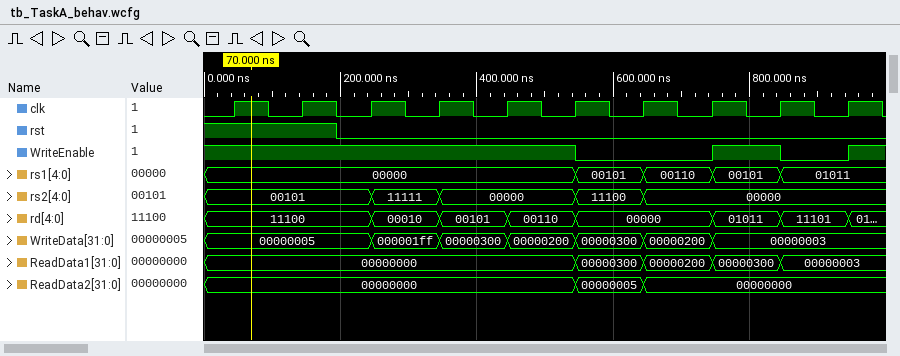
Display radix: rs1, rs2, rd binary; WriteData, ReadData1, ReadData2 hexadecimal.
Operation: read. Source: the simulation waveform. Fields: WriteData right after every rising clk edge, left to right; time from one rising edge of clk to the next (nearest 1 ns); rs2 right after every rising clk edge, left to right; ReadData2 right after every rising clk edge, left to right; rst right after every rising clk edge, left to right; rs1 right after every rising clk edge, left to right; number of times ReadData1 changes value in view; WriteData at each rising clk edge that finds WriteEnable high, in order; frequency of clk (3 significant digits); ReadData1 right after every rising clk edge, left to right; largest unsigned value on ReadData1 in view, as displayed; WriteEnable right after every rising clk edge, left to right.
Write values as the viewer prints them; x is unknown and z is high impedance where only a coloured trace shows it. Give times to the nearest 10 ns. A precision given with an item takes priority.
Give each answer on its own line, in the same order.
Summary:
00000005, 00000005, 000001ff, 00000300, 00000200, 00000300, 00000200, 00000003, 00000003, 00000003
100 ns
00101, 00101, 11111, 00000, 00000, 11100, 00000, 00000, 00000, 00000
00000000, 00000000, 00000000, 00000000, 00000000, 00000005, 00000000, 00000000, 00000000, 00000000
1 1 0 0 0 0 0 0 0 0
00000, 00000, 00000, 00000, 00000, 00101, 00110, 00101, 01011, 01011
4
00000005, 00000005, 00000005, 000001ff, 00000300, 00000200, 00000003
10.0 MHz
00000000, 00000000, 00000000, 00000000, 00000000, 00000300, 00000200, 00000300, 00000003, 00000003
00000300
1 1 1 1 1 0 0 1 0 1
